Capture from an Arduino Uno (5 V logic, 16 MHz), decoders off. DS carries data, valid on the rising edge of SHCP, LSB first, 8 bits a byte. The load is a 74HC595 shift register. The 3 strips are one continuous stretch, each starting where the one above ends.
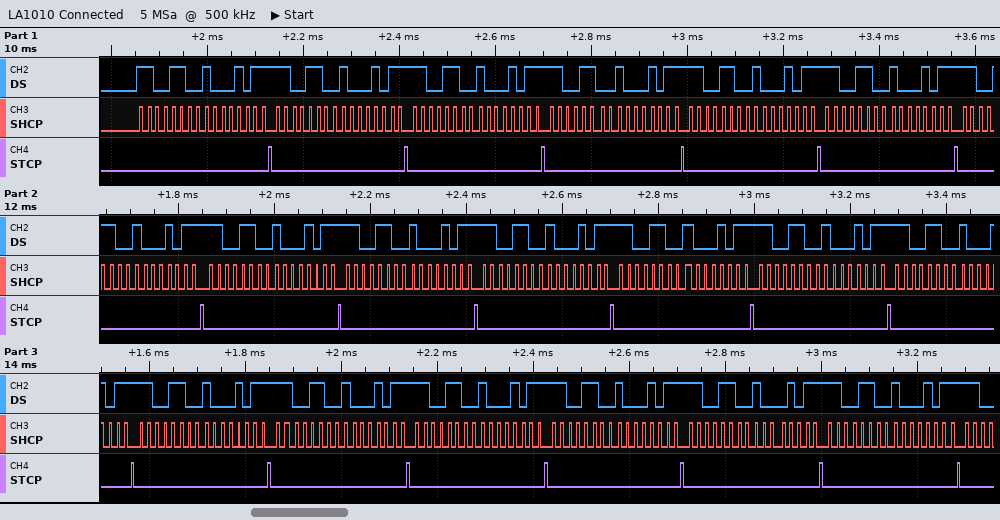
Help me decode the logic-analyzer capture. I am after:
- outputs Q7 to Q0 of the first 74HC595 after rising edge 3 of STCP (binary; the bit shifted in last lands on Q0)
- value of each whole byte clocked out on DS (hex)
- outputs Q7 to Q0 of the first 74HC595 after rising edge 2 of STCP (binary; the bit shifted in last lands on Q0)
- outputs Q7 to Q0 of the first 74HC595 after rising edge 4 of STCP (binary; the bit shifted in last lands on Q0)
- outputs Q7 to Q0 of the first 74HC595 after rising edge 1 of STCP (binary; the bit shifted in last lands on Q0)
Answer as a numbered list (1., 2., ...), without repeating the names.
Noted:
1. 10001011
2. 0x33 0xD1 0x33 0xD1 0x33 0xD1 0x33 0xD1 0x33 0xD1 0x33 0xD1 0x33 0xD1 0x33 0xD1 0x33 0xD1 0x33 0xD1 0x33 0xD1 0x33 0xD1 0x33 0xD1 0x33 0xD1 0x33 0xD1 0x33 0xD1 0x33 0xD1 0x33 0xD1 0x33 0xD1
3. 10001011
4. 10001011
5. 10001011
